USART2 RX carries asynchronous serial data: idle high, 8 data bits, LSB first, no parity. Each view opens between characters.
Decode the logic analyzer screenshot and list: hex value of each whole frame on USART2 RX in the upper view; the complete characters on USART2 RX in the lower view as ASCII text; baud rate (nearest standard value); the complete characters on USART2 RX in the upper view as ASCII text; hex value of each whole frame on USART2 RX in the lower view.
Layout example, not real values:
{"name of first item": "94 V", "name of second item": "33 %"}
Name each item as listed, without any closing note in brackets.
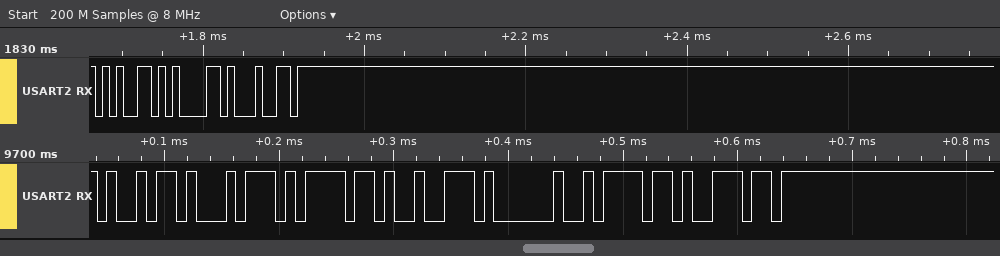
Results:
{"hex value of each whole frame on USART2 RX in the upper view": "65, 61, 64", "the complete characters on USART2 RX in the lower view as ASCII text": "\"itor on\"", "baud rate": "115200 baud", "the complete characters on USART2 RX in the upper view as ASCII text": "\"ead\"", "hex value of each whole frame on USART2 RX in the lower view": "69, 74, 6F, 72, 20, 6F, 6E"}
